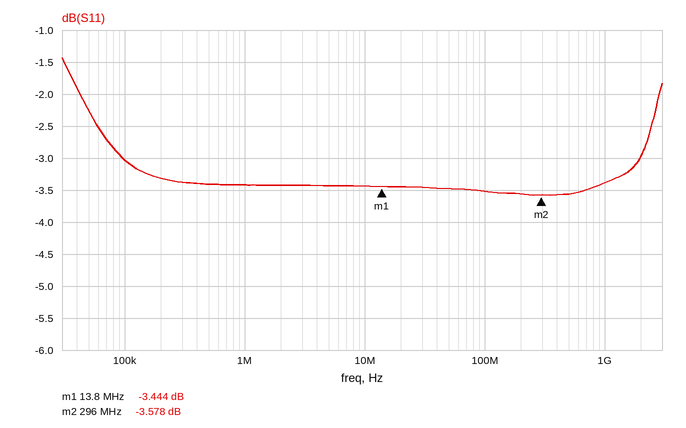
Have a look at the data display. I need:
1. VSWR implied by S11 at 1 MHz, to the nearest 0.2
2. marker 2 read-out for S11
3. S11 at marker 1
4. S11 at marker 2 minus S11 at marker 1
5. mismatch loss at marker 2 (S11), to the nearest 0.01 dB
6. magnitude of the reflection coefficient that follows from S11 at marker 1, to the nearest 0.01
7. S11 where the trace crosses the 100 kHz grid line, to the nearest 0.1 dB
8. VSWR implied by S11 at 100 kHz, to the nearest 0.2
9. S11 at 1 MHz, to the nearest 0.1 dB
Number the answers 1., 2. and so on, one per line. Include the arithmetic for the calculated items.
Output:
1. |Γ| = 10^(-3.4/20) = 0.6761; VSWR = (1 + 0.6761)/(1 − 0.6761) ≈ 5.2
2. -3.578 dB
3. -3.444 dB
4. -3.578 − (-3.444) = -0.134 dB
5. −10 log10(1 − 10^(-3.578/10)) ≈ 2.51 dB
6. 10^(-3.444/20) ≈ 0.67
7. -3.0 dB
8. |Γ| = 10^(-3/20) = 0.7079; VSWR = (1 + 0.7079)/(1 − 0.7079) ≈ 5.8
9. -3.4 dB
